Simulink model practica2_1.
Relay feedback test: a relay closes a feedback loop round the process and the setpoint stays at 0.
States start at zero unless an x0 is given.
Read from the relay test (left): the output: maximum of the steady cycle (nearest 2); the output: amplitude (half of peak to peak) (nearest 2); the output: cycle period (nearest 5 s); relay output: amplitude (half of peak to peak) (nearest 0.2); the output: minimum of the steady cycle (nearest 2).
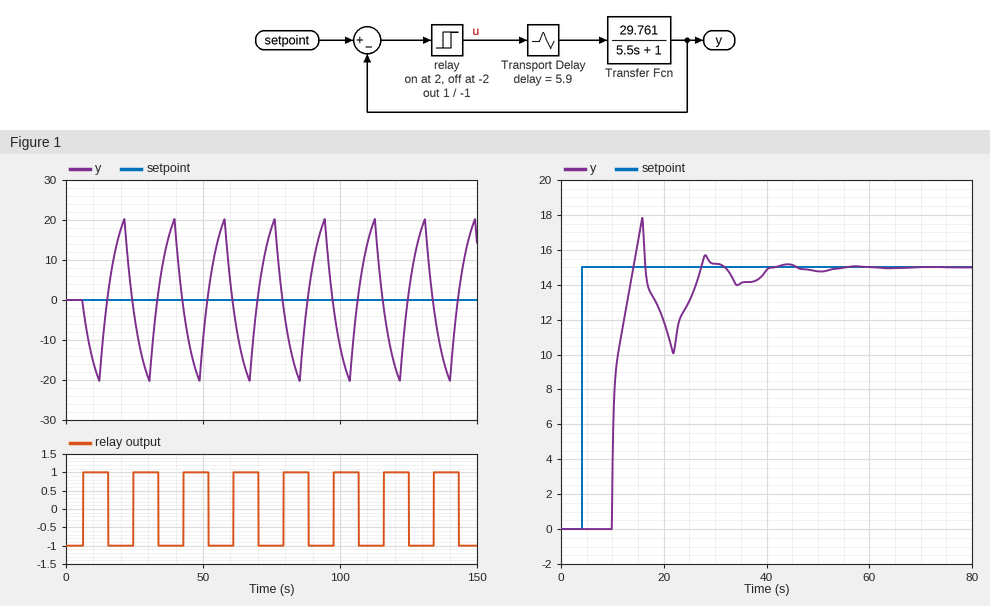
20
20
20 s
1.0
-20
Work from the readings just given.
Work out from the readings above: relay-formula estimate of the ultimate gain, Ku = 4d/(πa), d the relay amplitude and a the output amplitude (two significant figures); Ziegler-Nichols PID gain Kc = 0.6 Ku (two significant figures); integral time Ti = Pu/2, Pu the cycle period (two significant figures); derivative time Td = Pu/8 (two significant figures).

0.064
0.038
10 s
2.5 s
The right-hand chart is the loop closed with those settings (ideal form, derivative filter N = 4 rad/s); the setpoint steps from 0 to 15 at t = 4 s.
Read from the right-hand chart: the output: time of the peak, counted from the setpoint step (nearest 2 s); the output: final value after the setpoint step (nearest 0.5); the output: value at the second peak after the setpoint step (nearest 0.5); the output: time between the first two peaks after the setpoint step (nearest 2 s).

12 s
15.0
15.5
12 s
